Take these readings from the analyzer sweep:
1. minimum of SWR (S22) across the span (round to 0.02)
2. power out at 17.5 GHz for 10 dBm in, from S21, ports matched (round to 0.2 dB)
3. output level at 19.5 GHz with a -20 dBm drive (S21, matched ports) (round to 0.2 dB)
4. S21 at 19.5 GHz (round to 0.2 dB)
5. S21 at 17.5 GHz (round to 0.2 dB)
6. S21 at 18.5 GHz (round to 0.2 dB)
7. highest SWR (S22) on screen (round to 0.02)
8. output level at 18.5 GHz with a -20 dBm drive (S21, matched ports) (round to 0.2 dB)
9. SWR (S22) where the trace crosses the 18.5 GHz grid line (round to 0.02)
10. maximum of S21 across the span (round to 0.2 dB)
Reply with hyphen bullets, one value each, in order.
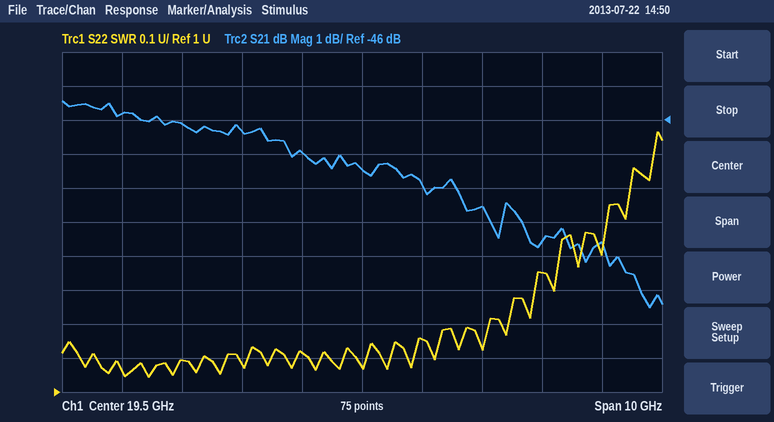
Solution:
- 1.04
- -36.4 dBm
- -67.4 dBm
- -47.4 dB
- -46.4 dB
- -47.0 dB
- 1.76
- -67.0 dBm
- 1.12
- -45.4 dB
